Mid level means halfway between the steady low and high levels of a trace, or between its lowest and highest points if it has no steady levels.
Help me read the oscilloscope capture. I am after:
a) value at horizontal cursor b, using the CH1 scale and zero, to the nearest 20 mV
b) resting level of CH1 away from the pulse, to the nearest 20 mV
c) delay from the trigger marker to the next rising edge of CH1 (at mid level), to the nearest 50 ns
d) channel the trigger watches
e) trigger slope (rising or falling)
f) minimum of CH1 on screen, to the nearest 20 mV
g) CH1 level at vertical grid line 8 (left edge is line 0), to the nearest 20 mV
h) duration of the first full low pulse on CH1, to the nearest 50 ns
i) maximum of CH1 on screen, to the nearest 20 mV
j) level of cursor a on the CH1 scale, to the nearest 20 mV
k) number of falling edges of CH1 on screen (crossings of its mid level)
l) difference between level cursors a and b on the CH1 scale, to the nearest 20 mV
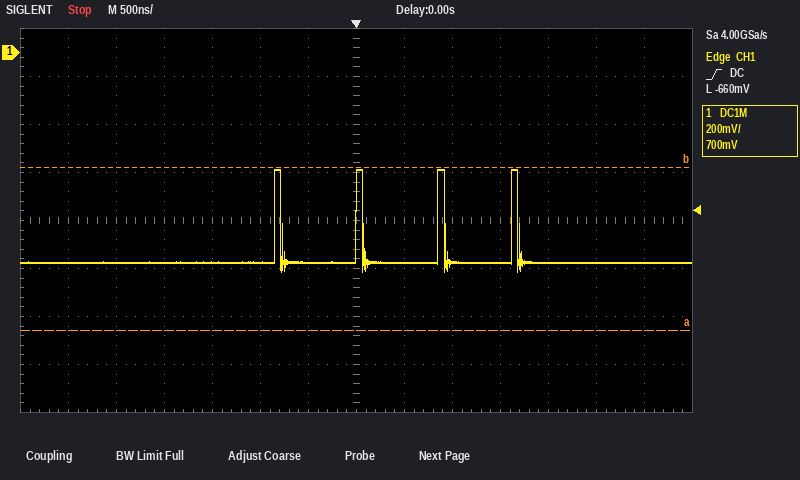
-480 mV
-880 mV
850 ns
CH1
rising
-920 mV
-880 mV
800 ns
-480 mV
-1.16 V
4
680 mV
